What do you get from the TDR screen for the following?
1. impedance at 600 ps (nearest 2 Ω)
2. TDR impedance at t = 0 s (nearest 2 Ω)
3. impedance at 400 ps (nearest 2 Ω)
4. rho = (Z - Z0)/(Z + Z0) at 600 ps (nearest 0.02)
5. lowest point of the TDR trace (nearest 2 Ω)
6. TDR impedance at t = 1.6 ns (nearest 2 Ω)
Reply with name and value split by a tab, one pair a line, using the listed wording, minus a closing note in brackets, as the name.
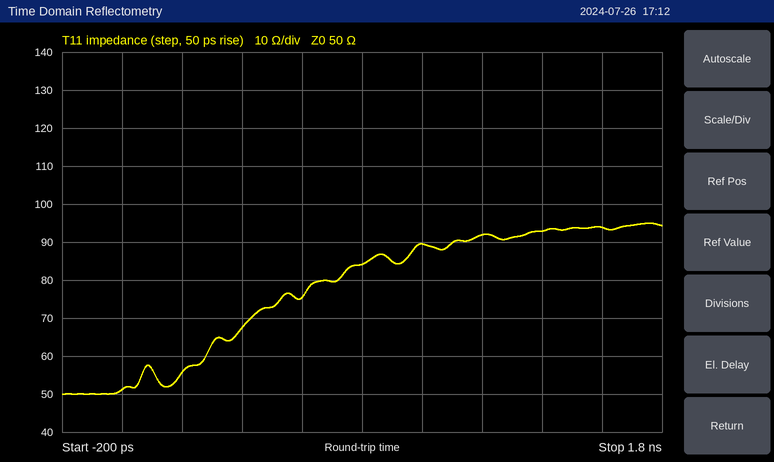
impedance at 600 ps	76 Ω
TDR impedance at t = 0 s	52 Ω
impedance at 400 ps	68 Ω
rho = (Z - Z0)/(Z + Z0) at 600 ps	+0.20
lowest point of the TDR trace	50 Ω
TDR impedance at t = 1.6 ns	94 Ω
